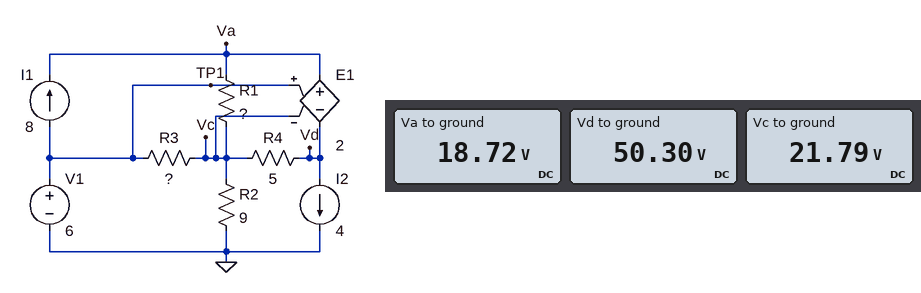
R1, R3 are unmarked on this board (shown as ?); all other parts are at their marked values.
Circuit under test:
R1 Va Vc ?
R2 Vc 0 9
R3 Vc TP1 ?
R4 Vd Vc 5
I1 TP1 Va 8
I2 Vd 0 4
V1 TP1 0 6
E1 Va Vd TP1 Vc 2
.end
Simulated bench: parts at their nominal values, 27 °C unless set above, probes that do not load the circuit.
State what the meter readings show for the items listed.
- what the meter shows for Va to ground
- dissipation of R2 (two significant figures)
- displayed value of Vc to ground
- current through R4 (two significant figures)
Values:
18.72 V
53 W
21.79 V
5.7 A
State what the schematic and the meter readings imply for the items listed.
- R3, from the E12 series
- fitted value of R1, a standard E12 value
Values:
10 Ω
1.8 Ω
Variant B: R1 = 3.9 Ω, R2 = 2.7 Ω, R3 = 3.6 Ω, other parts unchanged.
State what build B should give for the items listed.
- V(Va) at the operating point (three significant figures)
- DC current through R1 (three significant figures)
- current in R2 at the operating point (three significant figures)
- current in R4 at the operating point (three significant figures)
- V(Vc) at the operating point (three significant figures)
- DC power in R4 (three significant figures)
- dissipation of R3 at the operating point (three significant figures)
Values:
15.1 V
1.63 A
3.24 A
2.37 A
8.74 V
28.1 W
2.09 W
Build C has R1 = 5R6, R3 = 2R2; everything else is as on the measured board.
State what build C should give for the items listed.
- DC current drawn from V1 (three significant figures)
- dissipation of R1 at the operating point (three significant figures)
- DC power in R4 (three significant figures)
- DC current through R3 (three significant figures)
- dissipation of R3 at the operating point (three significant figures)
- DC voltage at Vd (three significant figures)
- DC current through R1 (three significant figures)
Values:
5.32 A
3.36 W
52.0 W
2.68 A
15.8 W
28.0 V
775 mA
